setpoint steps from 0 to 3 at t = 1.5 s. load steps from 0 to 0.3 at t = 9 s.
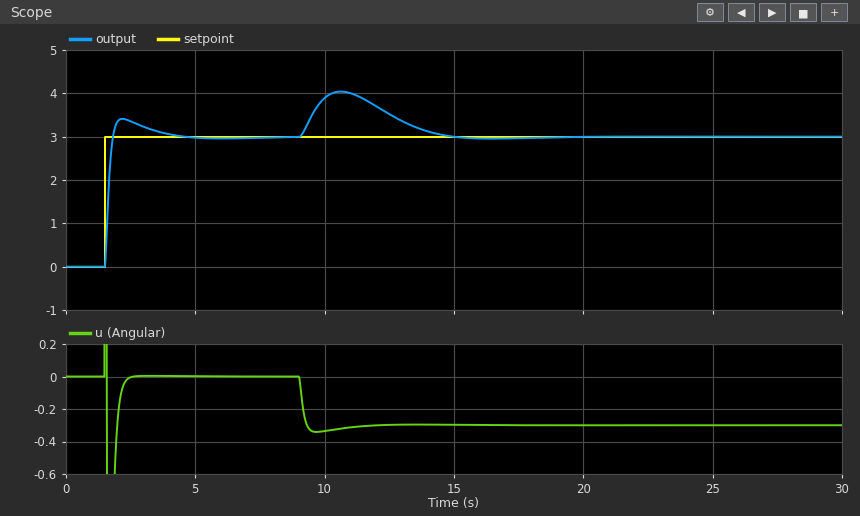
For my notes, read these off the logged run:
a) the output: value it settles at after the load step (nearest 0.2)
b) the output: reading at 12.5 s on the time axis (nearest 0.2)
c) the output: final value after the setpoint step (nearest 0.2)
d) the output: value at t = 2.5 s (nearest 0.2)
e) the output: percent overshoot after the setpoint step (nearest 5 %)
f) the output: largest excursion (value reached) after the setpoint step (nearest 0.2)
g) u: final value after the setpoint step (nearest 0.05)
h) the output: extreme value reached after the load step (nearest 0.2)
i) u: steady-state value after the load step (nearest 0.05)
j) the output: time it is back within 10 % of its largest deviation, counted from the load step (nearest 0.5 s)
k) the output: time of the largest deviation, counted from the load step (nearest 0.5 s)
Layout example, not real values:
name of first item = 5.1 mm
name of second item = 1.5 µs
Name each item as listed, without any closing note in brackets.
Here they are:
the output: value it settles at after the load step = 3.0
the output: reading at 12.5 s on the time axis = 3.6
the output: final value after the setpoint step = 3.0
the output: value at t = 2.5 s = 3.4
the output: percent overshoot after the setpoint step = 15 %
the output: largest excursion (value reached) after the setpoint step = 3.4
u: final value after the setpoint step = 0.00
the output: extreme value reached after the load step = 4.0
u: steady-state value after the load step = -0.30
the output: time it is back within 10 % of its largest deviation, counted from the load step = 5.0 s
the output: time of the largest deviation, counted from the load step = 1.5 s
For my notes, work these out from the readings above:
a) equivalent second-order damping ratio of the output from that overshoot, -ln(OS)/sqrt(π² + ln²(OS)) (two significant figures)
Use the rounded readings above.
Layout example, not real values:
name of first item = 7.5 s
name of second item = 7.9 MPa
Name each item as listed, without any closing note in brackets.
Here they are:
equivalent second-order damping ratio of the output from that overshoot, -ln(OS)/sqrt(π² + ln²(OS)) = 0.52
